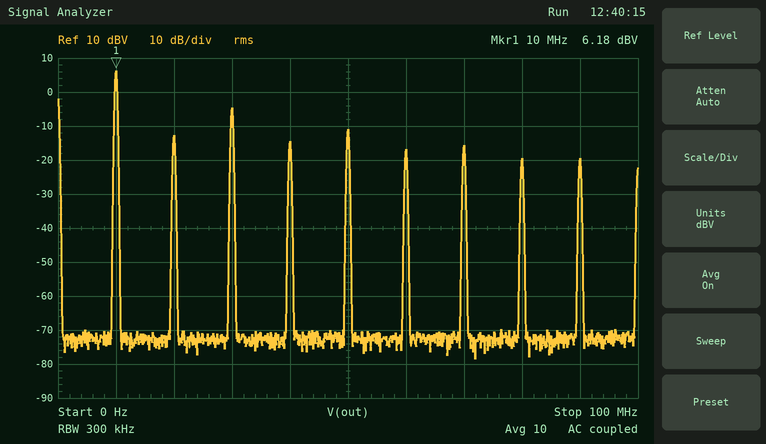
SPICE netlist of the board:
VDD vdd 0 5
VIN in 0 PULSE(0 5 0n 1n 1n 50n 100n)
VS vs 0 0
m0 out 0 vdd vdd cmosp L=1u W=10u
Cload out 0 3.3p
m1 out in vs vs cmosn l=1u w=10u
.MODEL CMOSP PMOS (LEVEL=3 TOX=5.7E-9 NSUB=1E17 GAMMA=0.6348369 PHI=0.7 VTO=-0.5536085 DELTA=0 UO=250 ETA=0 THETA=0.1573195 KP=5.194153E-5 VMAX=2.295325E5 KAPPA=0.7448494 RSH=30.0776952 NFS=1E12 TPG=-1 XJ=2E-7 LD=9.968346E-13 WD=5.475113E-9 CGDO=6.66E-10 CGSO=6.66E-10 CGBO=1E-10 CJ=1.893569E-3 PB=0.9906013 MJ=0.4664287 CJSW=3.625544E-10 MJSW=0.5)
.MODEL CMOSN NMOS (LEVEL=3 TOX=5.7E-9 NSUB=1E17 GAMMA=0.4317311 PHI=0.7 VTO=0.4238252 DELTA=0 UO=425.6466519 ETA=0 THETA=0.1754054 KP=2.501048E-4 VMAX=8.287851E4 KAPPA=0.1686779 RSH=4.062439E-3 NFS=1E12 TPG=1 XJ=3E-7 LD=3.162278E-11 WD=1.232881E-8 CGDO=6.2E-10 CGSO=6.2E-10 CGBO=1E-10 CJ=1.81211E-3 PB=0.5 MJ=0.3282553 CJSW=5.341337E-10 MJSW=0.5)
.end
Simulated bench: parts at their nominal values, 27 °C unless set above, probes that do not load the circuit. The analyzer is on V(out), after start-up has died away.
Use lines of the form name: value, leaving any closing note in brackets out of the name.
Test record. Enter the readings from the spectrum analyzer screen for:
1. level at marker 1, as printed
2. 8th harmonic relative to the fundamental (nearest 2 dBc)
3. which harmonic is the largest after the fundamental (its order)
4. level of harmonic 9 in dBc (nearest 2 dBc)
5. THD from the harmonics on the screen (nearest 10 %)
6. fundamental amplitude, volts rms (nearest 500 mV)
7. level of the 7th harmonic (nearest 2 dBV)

level at marker 1, as printed: 6.18 dBV
8th harmonic relative to the fundamental: -26 dBc
which harmonic is the largest after the fundamental: 3
level of harmonic 9 in dBc: -26 dBc
THD from the harmonics on the screen: 40 %
fundamental amplitude, volts rms: 2.0 V
level of the 7th harmonic: -16 dBV
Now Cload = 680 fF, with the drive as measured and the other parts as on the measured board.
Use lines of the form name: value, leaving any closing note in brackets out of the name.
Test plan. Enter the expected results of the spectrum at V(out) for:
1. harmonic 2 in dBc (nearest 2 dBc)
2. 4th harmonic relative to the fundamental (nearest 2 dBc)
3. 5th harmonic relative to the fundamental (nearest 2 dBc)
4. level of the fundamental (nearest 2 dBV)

harmonic 2 in dBc: -26 dBc
4th harmonic relative to the fundamental: -26 dBc
5th harmonic relative to the fundamental: -14 dBc
level of the fundamental: 6 dBV
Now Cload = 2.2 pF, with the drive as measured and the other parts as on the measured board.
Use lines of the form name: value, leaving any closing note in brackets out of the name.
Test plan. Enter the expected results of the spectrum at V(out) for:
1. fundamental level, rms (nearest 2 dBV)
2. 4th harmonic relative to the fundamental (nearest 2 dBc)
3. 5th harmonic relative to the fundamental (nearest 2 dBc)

fundamental level, rms: 6 dBV
4th harmonic relative to the fundamental: -22 dBc
5th harmonic relative to the fundamental: -16 dBc
